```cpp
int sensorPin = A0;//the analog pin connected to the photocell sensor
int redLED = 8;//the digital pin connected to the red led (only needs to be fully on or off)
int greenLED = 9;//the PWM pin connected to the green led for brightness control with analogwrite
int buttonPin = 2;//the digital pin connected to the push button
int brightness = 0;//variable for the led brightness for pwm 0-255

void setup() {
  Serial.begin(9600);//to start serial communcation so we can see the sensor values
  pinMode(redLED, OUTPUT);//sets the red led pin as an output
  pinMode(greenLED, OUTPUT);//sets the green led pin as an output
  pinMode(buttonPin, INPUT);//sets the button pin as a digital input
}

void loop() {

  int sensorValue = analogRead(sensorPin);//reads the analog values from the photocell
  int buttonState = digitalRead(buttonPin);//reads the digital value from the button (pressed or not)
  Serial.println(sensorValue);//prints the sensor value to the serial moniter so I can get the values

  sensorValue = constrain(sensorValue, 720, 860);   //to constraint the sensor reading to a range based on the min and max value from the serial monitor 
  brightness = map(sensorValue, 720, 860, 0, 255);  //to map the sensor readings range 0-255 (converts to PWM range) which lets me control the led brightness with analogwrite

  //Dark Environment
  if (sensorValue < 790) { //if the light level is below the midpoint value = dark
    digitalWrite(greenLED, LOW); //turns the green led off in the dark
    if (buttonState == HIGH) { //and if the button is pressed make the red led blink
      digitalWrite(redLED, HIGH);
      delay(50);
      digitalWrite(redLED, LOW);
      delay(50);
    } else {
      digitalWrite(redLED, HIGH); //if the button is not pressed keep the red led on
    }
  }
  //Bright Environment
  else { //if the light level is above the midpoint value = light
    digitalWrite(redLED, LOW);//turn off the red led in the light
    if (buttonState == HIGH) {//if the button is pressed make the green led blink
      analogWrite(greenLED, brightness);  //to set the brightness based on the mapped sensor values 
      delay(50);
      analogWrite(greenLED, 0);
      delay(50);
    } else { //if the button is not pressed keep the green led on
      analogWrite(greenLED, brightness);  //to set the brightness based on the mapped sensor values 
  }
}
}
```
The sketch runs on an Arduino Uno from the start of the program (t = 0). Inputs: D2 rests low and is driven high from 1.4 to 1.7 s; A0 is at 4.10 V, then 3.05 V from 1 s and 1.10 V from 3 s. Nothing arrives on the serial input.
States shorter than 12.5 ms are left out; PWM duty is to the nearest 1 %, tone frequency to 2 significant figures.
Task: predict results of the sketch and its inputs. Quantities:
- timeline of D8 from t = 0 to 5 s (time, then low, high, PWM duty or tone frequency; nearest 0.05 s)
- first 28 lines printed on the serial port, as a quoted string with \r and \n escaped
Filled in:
0 s low; 1 s high; 1.45 s low; 1.5 s high; 1.55 s low; 1.6 s high; 1.65 s low; 1.7 s high
"839\r\n839\r\n839\r\n839\r\n839\r\n839\r\n839\r\n839\r\n839\r\n839\r\n839\r\n839\r\n839\r\n839\r\n839\r\n839\r\n839\r\n839\r\n839\r\n839\r\n839\r\n839\r\n839\r\n839\r\n839\r\n839\r\n839\r\n839\r\n"
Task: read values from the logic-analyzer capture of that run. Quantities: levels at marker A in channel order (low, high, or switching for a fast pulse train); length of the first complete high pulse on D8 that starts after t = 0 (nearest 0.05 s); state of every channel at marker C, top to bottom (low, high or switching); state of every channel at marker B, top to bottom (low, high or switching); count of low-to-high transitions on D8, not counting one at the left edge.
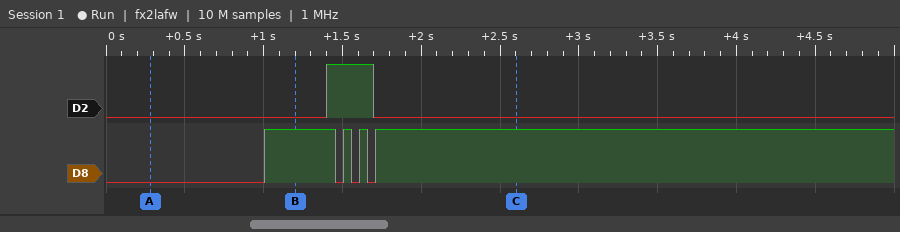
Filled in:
D2 low, D8 low
0.45 s
D2 low, D8 high
D2 low, D8 high
4
